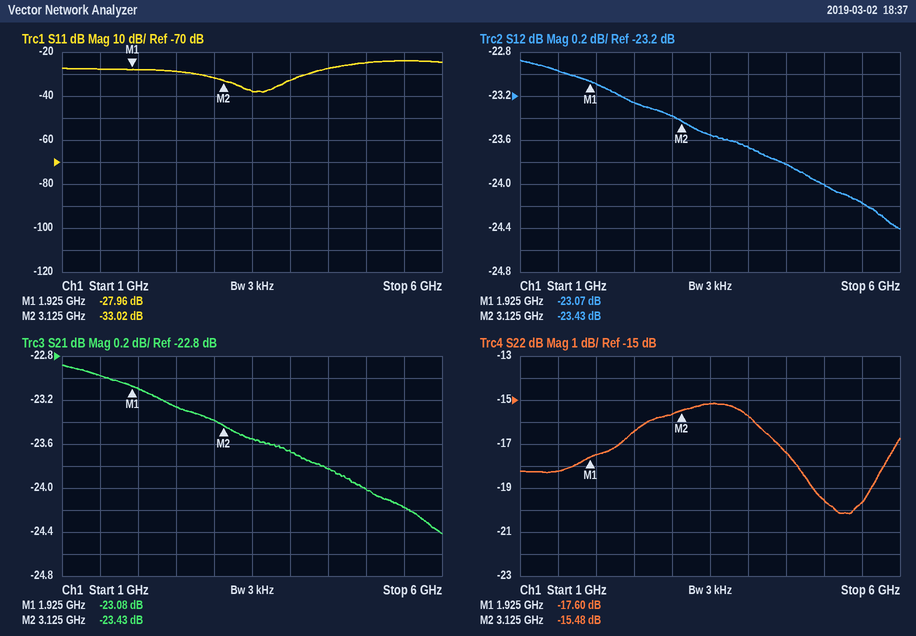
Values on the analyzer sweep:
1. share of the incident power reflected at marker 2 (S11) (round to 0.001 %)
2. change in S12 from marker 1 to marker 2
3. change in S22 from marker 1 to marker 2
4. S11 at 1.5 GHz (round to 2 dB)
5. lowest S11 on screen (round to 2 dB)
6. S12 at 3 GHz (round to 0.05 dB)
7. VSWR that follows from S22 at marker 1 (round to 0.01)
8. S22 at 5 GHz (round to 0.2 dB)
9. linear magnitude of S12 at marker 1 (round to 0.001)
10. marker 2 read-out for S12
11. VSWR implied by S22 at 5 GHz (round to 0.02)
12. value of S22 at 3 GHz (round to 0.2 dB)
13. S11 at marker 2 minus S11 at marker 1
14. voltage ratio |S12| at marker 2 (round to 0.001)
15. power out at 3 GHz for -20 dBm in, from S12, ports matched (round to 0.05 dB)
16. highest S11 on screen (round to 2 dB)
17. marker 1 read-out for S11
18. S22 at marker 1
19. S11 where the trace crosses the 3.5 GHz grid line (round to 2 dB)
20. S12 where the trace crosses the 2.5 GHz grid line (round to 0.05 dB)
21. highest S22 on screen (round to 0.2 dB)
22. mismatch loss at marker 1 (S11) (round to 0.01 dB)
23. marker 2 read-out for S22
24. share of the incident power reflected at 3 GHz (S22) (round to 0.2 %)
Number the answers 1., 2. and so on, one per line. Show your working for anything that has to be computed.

1. 10^(-33.02/10) ≈ 0.050 %
2. -23.43 − (-23.07) = -0.36 dB
3. -15.48 − (-17.6) = 2.12 dB
4. -28 dB
5. -38 dB
6. -23.40 dB
7. (1 + 0.1318)/(1 − 0.1318) ≈ 1.30
8. -19.6 dB
9. 10^(-23.07/20) ≈ 0.070
10. -23.43 dB
11. |Γ| = 10^(-19.6/20) = 0.1047; VSWR = (1 + 0.1047)/(1 − 0.1047) ≈ 1.23, so 1.24 to the nearest 0.02
12. -15.6 dB
13. -33.02 − (-27.96) = -5.06 dB
14. 10^(-23.43/20) ≈ 0.067
15. -20 dBm + (-23.40 dB) = -43.40 dBm
16. -24 dB
17. -27.96 dB
18. -17.60 dB
19. -38 dB
20. -23.25 dB
21. -15.2 dB
22. −10 log10(1 − 10^(-27.96/10)) ≈ 0.01 dB
23. -15.48 dB
24. 10^(-15.6/10) ≈ 2.8 %
